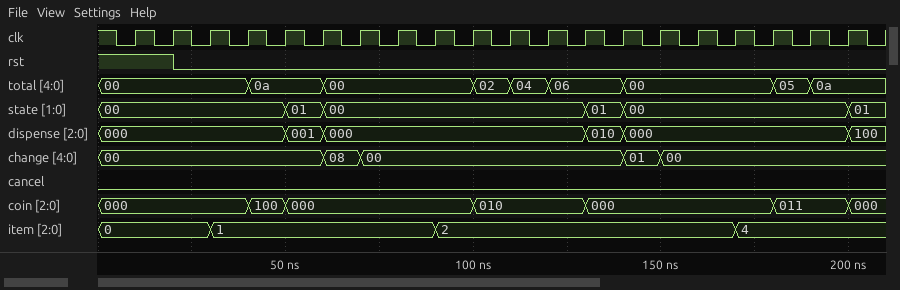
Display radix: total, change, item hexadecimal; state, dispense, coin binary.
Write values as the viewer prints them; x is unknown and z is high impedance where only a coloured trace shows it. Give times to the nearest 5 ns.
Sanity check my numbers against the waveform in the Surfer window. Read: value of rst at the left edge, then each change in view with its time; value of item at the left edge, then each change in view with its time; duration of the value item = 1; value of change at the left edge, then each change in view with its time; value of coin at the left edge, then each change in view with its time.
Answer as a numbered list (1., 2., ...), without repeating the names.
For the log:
1. 1, 0 at 20 ns
2. 0, 1 at 30 ns, 2 at 90 ns, 4 at 170 ns
3. 60 ns
4. 00, 08 at 60 ns, 00 at 70 ns, 01 at 140 ns, 00 at 150 ns
5. 000, 100 at 40 ns, 000 at 50 ns, 010 at 100 ns, 000 at 130 ns, 011 at 180 ns, 000 at 200 ns
